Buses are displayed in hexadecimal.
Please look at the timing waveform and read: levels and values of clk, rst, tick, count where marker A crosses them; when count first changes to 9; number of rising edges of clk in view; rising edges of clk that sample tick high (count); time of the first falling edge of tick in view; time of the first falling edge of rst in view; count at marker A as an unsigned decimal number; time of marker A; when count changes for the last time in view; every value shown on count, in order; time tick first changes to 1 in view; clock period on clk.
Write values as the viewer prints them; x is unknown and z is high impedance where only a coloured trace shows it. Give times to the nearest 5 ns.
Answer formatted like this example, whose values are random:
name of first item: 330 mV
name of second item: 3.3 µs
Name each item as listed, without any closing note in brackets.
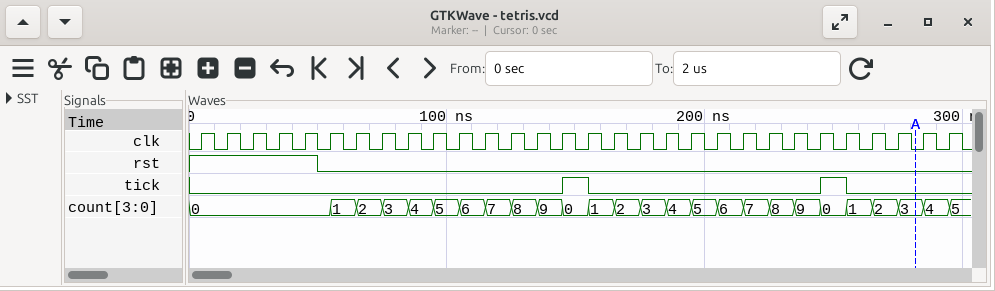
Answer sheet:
levels and values of clk, rst, tick, count where marker A crosses them: clk=0, rst=0, tick=0, count=3
when count first changes to 9: 135 ns
number of rising edges of clk in view: 30
rising edges of clk that sample tick high: 2
time of the first falling edge of tick in view: 155 ns
time of the first falling edge of rst in view: 50 ns
count at marker A as an unsigned decimal number: 3
time of marker A: 280 ns
when count changes for the last time in view: 295 ns
every value shown on count, in order: 0, 1, 2, 3, 4, 5, 6, 7, 8, 9, 0, 1, 2, 3, 4, 5, 6, 7, 8, 9, 0, 1, 2, 3, 4, 5
time tick first changes to 1 in view: 145 ns
clock period on clk: 10 ns
